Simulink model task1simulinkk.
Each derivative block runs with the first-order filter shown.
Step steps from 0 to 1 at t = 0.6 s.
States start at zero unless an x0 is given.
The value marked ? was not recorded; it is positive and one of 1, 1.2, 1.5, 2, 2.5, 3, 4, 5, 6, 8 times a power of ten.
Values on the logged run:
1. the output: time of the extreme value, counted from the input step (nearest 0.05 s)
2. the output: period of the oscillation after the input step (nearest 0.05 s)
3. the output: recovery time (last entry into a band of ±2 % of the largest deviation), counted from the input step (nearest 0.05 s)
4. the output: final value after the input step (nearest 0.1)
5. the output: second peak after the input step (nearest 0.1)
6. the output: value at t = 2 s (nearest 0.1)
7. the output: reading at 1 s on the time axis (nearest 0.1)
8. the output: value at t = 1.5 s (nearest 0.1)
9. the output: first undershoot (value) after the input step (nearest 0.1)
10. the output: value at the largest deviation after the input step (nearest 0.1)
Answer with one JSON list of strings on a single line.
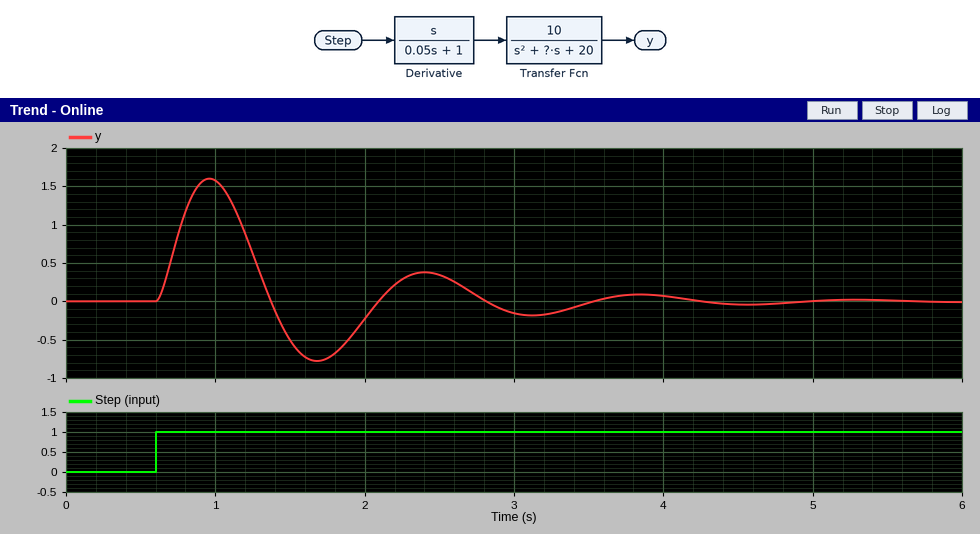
["0.35 s", "1.45 s", "4.15 s", "0.0", "0.4", "-0.2", "1.6", "-0.5", "-0.8", "1.6"]
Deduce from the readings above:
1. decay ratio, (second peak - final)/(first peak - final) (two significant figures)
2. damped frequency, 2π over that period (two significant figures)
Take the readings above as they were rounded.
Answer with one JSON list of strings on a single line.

["0.25", "4.3 rad/s"]
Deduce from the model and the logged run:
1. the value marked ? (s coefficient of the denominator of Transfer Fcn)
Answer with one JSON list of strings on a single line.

["2"]
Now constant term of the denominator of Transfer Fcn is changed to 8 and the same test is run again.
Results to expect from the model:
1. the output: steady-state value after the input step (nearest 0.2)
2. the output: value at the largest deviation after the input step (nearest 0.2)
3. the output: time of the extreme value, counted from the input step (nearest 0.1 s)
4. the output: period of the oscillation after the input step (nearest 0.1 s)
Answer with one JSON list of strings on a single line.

["0.0", "2.2", "0.5 s", "2.4 s"]
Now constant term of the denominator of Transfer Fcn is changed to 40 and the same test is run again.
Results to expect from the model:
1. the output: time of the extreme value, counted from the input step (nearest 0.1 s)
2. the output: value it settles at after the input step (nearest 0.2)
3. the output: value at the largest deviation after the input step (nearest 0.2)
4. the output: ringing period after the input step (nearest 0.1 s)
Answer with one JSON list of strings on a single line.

["0.3 s", "0.0", "1.2", "1.0 s"]
